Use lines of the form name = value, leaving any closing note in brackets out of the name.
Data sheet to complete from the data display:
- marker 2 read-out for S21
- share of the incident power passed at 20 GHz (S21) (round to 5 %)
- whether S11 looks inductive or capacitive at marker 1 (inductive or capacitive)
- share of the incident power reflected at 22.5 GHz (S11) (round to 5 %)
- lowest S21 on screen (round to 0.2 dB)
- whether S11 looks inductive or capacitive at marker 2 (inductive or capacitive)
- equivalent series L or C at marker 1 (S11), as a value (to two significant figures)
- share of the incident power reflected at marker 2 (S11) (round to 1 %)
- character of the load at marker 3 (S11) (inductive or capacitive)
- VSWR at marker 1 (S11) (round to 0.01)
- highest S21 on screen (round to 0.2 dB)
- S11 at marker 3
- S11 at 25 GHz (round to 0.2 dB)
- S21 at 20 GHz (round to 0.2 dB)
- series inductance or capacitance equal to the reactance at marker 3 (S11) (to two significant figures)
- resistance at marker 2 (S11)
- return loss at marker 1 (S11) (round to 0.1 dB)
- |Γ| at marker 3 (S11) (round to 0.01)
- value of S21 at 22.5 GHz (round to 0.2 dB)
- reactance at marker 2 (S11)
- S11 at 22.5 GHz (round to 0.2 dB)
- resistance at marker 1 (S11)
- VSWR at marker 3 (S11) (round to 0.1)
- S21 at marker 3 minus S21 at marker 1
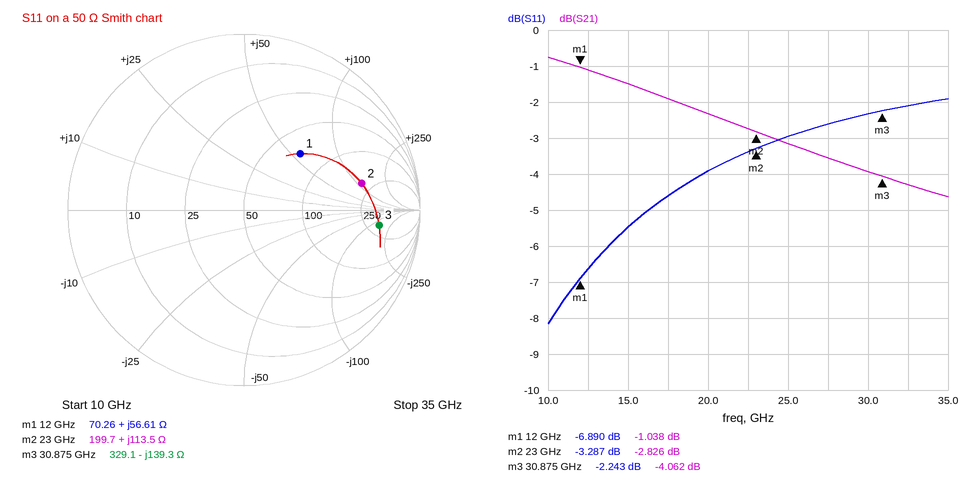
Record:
marker 2 read-out for S21 = -2.826 dB
share of the incident power passed at 20 GHz (S21) = 60 %
whether S11 looks inductive or capacitive at marker 1 = inductive
share of the incident power reflected at 22.5 GHz (S11) = 45 %
lowest S21 on screen = -4.6 dB
whether S11 looks inductive or capacitive at marker 2 = inductive
equivalent series L or C at marker 1 (S11), as a value = 750 pH
share of the incident power reflected at marker 2 (S11) = 47 %
character of the load at marker 3 (S11) = capacitive
VSWR at marker 1 (S11) = 2.65
highest S21 on screen = -0.8 dB
S11 at marker 3 = -2.243 dB
S11 at 25 GHz = -3.0 dB
S21 at 20 GHz = -2.4 dB
series inductance or capacitance equal to the reactance at marker 3 (S11) = 37 fF
resistance at marker 2 = 199.7 Ω
return loss at marker 1 (S11) = 6.9 dB
|Γ| at marker 3 (S11) = 0.77
value of S21 at 22.5 GHz = -2.8 dB
reactance at marker 2 = +113.5 Ω
S11 at 22.5 GHz = -3.4 dB
resistance at marker 1 = 70.26 Ω
VSWR at marker 3 (S11) = 7.8
S21 at marker 3 minus S21 at marker 1 = -3.024 dB
